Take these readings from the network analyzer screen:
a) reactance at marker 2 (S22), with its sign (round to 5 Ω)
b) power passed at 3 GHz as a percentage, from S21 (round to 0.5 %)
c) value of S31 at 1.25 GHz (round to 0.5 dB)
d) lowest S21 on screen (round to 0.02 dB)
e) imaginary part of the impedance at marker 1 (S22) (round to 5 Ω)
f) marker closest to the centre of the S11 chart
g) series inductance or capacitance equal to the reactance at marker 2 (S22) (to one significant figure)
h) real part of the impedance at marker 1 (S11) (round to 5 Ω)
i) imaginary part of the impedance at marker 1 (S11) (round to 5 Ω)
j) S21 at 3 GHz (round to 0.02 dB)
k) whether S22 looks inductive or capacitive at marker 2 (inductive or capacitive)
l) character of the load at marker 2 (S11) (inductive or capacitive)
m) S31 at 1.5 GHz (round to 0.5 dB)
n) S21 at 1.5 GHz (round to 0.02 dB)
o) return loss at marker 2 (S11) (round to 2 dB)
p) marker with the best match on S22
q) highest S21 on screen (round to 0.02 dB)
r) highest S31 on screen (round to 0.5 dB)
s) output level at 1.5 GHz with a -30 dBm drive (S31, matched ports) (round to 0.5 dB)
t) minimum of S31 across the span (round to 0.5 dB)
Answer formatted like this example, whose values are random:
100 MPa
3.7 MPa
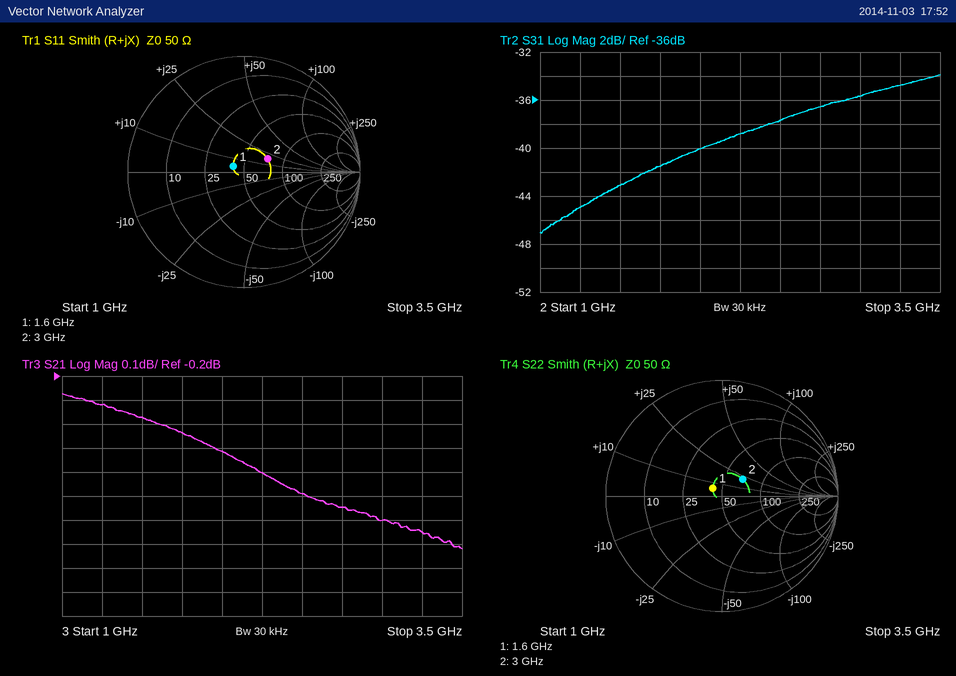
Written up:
+20 Ω
83.0 %
-45.0 dB
-0.92 dB
+5 Ω
marker 1
1 nH
40 Ω
+5 Ω
-0.80 dB
inductive
inductive
-43.0 dB
-0.38 dB
12 dB
marker 1
-0.28 dB
-34.0 dB
-73.0 dBm
-47.0 dB
